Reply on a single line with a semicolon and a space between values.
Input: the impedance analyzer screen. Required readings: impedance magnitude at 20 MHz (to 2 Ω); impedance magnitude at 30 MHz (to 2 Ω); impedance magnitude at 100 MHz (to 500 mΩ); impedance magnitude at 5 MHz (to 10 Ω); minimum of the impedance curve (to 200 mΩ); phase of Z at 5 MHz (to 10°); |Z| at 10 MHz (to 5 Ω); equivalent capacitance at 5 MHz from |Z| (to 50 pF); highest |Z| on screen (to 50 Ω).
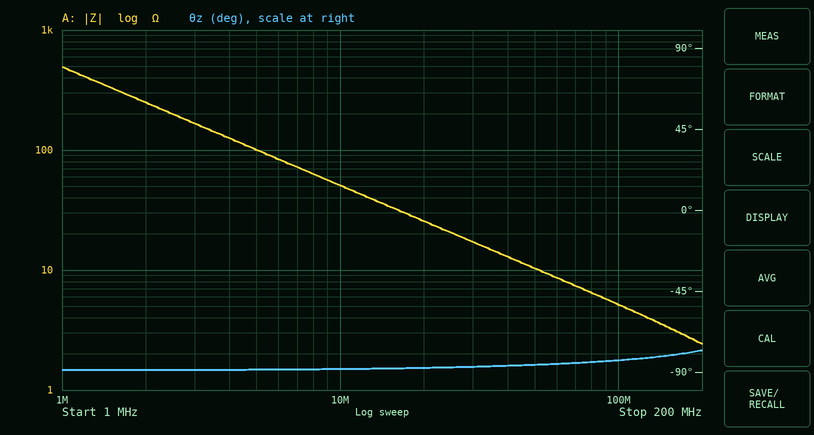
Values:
26 Ω; 18 Ω; 5.0 Ω; 100 Ω; 2.4 Ω; -90°; 50 Ω; 300 pF; 500 Ω
